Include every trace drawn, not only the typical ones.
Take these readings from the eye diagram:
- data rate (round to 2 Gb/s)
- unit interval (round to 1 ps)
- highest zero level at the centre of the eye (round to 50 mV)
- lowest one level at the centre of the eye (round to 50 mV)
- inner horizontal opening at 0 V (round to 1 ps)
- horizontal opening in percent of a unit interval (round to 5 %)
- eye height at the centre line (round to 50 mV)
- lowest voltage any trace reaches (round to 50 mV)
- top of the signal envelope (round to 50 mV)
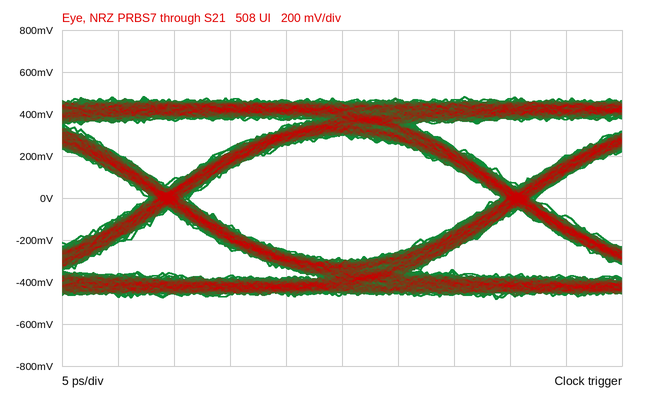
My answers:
32 Gb/s
31 ps
-300 mV
300 mV
28 ps
90 %
600 mV
-500 mV
500 mV
